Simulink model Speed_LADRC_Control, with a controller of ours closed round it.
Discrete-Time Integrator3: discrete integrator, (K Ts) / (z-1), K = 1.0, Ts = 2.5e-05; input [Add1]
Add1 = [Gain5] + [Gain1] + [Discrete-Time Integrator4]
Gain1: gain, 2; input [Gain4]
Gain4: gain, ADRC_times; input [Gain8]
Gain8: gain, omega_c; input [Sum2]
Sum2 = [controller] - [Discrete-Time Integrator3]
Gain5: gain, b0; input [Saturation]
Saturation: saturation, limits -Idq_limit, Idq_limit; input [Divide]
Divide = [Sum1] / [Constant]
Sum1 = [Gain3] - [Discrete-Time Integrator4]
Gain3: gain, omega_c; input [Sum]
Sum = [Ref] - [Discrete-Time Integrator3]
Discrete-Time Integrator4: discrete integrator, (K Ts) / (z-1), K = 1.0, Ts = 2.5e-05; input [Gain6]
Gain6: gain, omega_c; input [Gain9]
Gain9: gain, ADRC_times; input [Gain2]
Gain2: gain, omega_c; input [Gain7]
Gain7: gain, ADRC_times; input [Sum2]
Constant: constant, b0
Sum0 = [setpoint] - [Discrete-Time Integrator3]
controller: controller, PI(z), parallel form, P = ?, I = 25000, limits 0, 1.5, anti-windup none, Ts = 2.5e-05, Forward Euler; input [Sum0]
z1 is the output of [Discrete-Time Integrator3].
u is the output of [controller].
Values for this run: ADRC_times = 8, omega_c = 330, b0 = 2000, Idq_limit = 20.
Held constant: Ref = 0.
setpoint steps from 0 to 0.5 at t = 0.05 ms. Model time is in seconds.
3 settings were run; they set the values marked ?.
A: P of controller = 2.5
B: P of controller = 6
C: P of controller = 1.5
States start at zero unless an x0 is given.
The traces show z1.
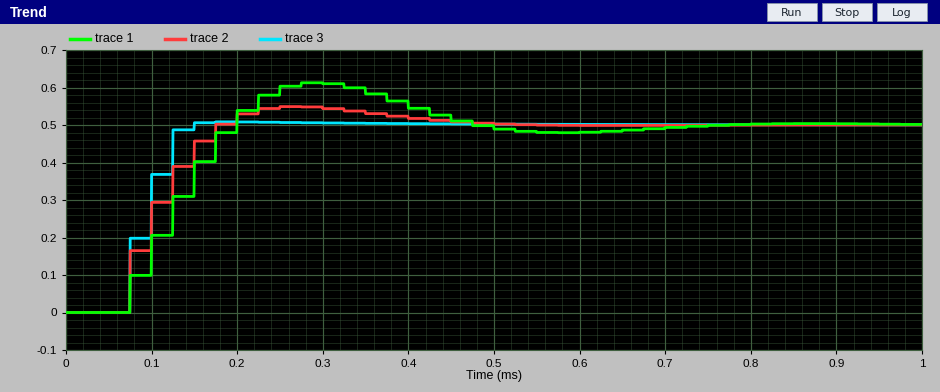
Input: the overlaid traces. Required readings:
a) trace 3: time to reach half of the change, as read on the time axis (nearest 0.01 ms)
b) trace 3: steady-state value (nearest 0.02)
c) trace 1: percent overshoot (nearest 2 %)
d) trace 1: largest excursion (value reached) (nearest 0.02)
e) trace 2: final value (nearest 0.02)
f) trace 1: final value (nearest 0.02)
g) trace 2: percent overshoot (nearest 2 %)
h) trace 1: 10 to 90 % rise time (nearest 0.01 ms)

0.10 ms
0.50
22 %
0.62
0.50
0.50
10 %
0.10 ms
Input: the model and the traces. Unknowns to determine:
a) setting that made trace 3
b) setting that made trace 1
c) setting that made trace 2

B
C
A
